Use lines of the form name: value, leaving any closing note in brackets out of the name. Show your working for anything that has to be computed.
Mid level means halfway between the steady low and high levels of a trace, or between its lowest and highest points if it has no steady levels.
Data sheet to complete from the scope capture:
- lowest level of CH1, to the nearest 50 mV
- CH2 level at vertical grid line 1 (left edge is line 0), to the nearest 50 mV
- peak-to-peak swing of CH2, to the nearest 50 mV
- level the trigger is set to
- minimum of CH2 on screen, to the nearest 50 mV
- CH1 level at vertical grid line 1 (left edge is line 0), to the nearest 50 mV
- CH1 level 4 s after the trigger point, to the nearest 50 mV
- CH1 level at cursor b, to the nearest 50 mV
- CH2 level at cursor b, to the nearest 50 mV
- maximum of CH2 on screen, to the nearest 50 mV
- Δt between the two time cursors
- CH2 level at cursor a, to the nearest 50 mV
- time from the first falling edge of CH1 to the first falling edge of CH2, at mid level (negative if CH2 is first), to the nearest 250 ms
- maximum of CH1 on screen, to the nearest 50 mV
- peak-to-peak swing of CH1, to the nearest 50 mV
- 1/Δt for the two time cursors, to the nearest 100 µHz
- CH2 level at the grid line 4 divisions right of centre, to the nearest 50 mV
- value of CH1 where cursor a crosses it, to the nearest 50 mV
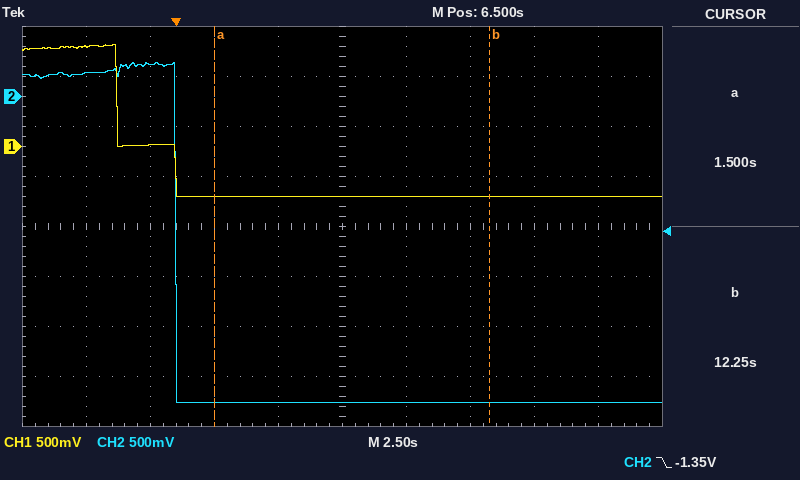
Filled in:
lowest level of CH1, to the nearest 50 mV: -500 mV
CH2 level at vertical grid line 1 (left edge is line 0), to the nearest 50 mV: 250 mV
peak-to-peak swing of CH2, to the nearest 50 mV: 350 mV − (-3.05 V) = 3.40 V
level the trigger is set to: -1.35 V
minimum of CH2 on screen, to the nearest 50 mV: -3.05 V
CH1 level at vertical grid line 1 (left edge is line 0), to the nearest 50 mV: 1.00 V
CH1 level 4 s after the trigger point, to the nearest 50 mV: -500 mV
CH1 level at cursor b, to the nearest 50 mV: -500 mV
CH2 level at cursor b, to the nearest 50 mV: -3.05 V
maximum of CH2 on screen, to the nearest 50 mV: 350 mV
Δt between the two time cursors: 12.25 s − (1.5 s) = 10.75 s
CH2 level at cursor a, to the nearest 50 mV: -3.05 V
time from the first falling edge of CH1 to the first falling edge of CH2, at mid level (negative if CH2 is first), to the nearest 250 ms: +2.25 s
maximum of CH1 on screen, to the nearest 50 mV: 1.00 V
peak-to-peak swing of CH1, to the nearest 50 mV: 1.00 V − (-500 mV) = 1.50 V
1/Δt for the two time cursors, to the nearest 100 µHz: 1 / 10.75 s ≈ 93.0 mHz
CH2 level at the grid line 4 divisions right of centre, to the nearest 50 mV: -3.05 V
value of CH1 where cursor a crosses it, to the nearest 50 mV: -500 mV
